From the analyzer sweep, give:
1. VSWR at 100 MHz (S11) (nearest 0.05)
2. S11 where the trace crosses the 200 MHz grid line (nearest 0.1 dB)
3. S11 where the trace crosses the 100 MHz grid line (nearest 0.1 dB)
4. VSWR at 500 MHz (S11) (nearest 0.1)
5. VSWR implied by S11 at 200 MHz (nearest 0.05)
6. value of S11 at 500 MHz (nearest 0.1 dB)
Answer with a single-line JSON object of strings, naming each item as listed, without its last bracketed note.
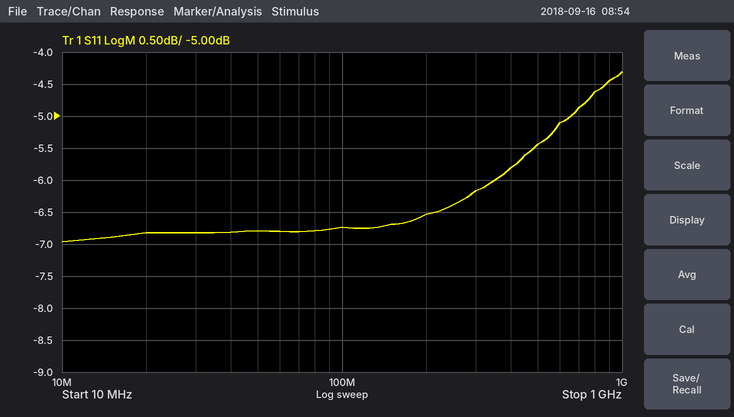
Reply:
{"VSWR at 100 MHz (S11)": "2.70", "S11 where the trace crosses the 200 MHz grid line": "-6.5 dB", "S11 where the trace crosses the 100 MHz grid line": "-6.7 dB", "VSWR at 500 MHz (S11)": "3.3", "VSWR implied by S11 at 200 MHz": "2.80", "value of S11 at 500 MHz": "-5.4 dB"}
